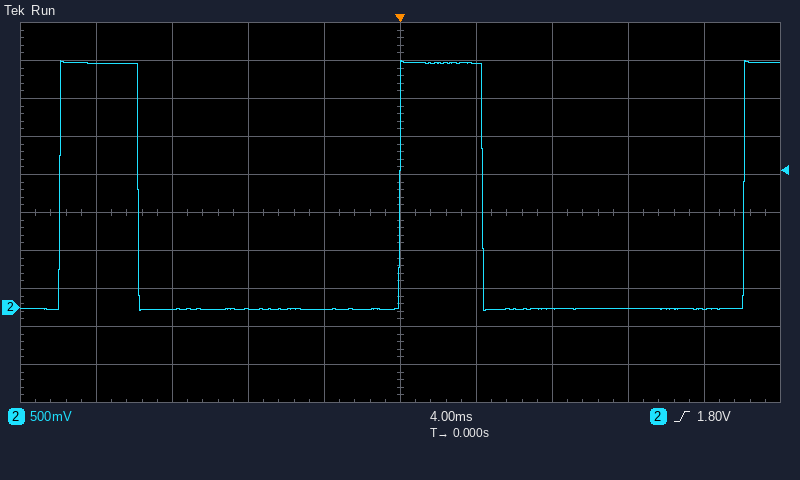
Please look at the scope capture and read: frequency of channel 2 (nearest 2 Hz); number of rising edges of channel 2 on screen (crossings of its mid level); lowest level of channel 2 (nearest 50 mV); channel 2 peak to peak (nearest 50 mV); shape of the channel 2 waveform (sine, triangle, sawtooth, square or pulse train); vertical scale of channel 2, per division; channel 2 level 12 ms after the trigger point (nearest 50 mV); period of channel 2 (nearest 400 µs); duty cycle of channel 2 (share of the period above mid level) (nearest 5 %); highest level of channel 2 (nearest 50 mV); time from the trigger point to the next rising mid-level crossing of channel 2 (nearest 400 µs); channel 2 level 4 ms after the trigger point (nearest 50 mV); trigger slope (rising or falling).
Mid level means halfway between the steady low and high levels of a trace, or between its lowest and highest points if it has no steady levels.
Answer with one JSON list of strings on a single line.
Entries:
["56 Hz", "3", "-50 mV", "3.30 V", "pulse train", "500 mV", "0 mV", "18.0 ms", "25 %", "3.25 V", "18.0 ms", "3.20 V", "rising"]
